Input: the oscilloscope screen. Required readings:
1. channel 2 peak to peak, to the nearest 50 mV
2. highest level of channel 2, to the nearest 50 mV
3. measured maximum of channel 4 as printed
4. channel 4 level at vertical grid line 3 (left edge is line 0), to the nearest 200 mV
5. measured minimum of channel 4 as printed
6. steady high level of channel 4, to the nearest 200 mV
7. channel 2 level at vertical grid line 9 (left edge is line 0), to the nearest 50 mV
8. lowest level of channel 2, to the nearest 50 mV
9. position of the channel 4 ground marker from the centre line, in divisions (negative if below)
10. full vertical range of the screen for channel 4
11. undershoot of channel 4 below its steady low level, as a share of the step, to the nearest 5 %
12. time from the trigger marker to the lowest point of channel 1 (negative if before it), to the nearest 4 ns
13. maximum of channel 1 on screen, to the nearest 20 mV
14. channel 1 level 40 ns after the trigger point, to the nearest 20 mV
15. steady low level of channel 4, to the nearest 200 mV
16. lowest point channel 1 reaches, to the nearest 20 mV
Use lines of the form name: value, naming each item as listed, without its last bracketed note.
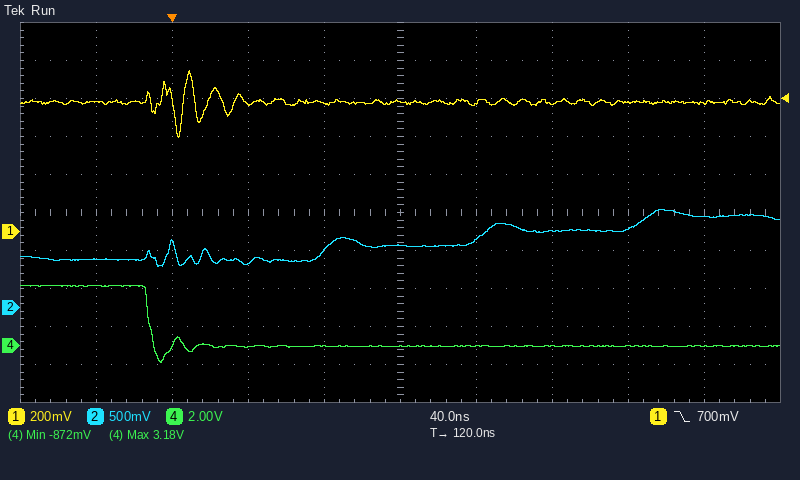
channel 2 peak to peak, to the nearest 50 mV: 750 mV
highest level of channel 2, to the nearest 50 mV: 1.30 V
measured maximum of channel 4 as printed: 3.18 V
channel 4 level at vertical grid line 3 (left edge is line 0), to the nearest 200 mV: 0.0 V
measured minimum of channel 4 as printed: -872 mV
steady high level of channel 4, to the nearest 200 mV: 3.2 V
channel 2 level at vertical grid line 9 (left edge is line 0), to the nearest 50 mV: 1.20 V
lowest level of channel 2, to the nearest 50 mV: 550 mV
position of the channel 4 ground marker from the centre line, in divisions: -3.5 div
full vertical range of the screen for channel 4: 20 V
undershoot of channel 4 below its steady low level, as a share of the step, to the nearest 5 %: 25 %
time from the trigger marker to the lowest point of channel 1 (negative if before it), to the nearest 4 ns: +4 ns
maximum of channel 1 on screen, to the nearest 20 mV: 840 mV
channel 1 level 40 ns after the trigger point, to the nearest 20 mV: 680 mV
steady low level of channel 4, to the nearest 200 mV: 0.0 V
lowest point channel 1 reaches, to the nearest 20 mV: 500 mV
